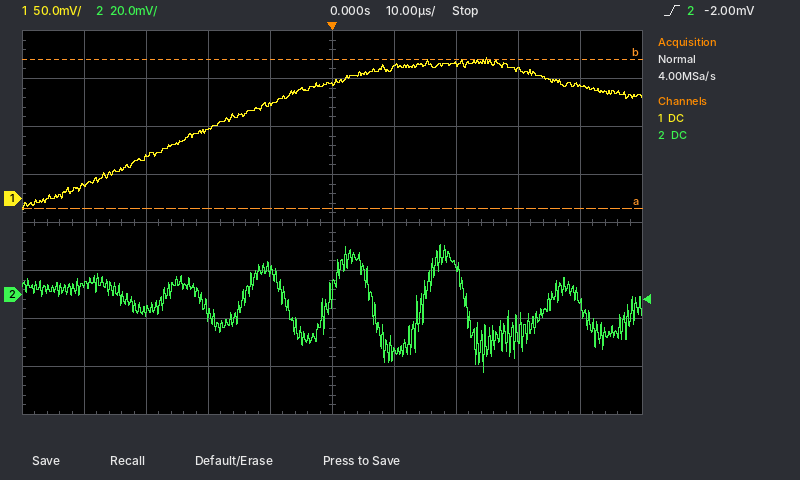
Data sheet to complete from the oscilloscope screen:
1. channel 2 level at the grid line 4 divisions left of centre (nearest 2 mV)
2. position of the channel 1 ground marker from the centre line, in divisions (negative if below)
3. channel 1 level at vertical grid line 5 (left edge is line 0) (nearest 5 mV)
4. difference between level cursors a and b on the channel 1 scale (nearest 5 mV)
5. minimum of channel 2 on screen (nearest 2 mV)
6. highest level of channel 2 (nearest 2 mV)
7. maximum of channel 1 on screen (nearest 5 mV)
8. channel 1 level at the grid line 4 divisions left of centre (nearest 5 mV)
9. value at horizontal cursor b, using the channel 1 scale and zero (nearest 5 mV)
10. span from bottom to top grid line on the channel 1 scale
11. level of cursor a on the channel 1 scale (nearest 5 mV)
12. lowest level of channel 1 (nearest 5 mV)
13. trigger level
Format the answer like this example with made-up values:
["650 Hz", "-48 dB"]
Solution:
["4 mV", "+0.5 div", "120 mV", "155 mV", "-32 mV", "20 mV", "145 mV", "15 mV", "145 mV", "400 mV", "-10 mV", "-10 mV", "-2.00 mV"]
